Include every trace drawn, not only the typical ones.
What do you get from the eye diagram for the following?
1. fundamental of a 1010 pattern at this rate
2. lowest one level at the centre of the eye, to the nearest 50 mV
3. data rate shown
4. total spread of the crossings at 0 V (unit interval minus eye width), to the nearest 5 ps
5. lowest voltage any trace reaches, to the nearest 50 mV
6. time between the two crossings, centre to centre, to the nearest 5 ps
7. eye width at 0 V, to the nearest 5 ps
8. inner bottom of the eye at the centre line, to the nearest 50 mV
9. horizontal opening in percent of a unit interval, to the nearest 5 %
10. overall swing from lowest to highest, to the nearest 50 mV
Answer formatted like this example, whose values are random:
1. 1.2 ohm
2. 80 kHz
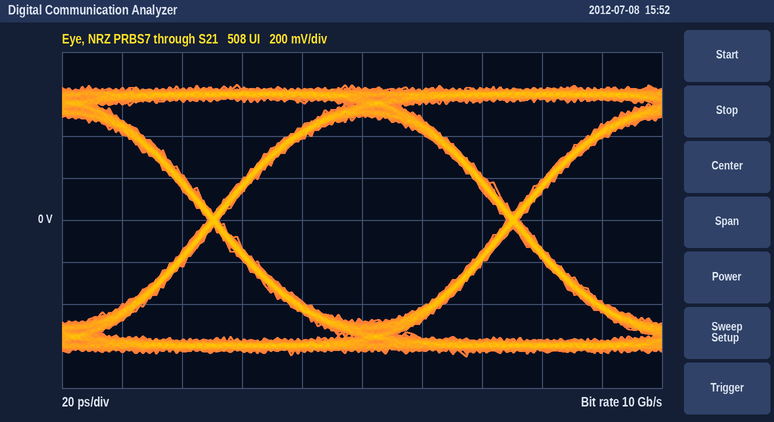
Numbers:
1. 5 GHz
2. 500 mV
3. 10 Gb/s
4. 5 ps
5. -650 mV
6. 100 ps
7. 95 ps
8. -500 mV
9. 95 %
10. 1.30 V
